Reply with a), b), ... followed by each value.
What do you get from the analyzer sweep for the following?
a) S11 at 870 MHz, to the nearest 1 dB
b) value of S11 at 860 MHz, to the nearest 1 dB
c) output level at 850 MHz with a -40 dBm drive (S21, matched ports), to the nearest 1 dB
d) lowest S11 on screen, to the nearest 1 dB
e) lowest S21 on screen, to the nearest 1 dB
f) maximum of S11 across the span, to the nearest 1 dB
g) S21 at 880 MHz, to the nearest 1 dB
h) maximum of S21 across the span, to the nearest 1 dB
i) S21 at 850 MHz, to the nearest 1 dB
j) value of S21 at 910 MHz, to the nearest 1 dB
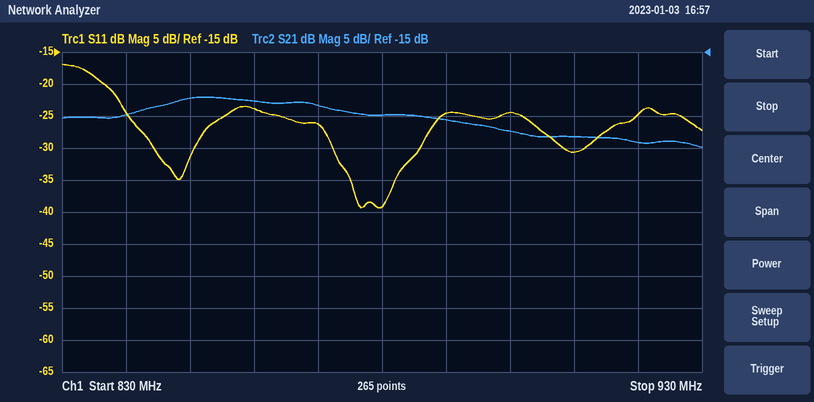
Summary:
a) -26 dB
b) -24 dB
c) -62 dBm
d) -39 dB
e) -30 dB
f) -17 dB
g) -25 dB
h) -22 dB
i) -22 dB
j) -28 dB
